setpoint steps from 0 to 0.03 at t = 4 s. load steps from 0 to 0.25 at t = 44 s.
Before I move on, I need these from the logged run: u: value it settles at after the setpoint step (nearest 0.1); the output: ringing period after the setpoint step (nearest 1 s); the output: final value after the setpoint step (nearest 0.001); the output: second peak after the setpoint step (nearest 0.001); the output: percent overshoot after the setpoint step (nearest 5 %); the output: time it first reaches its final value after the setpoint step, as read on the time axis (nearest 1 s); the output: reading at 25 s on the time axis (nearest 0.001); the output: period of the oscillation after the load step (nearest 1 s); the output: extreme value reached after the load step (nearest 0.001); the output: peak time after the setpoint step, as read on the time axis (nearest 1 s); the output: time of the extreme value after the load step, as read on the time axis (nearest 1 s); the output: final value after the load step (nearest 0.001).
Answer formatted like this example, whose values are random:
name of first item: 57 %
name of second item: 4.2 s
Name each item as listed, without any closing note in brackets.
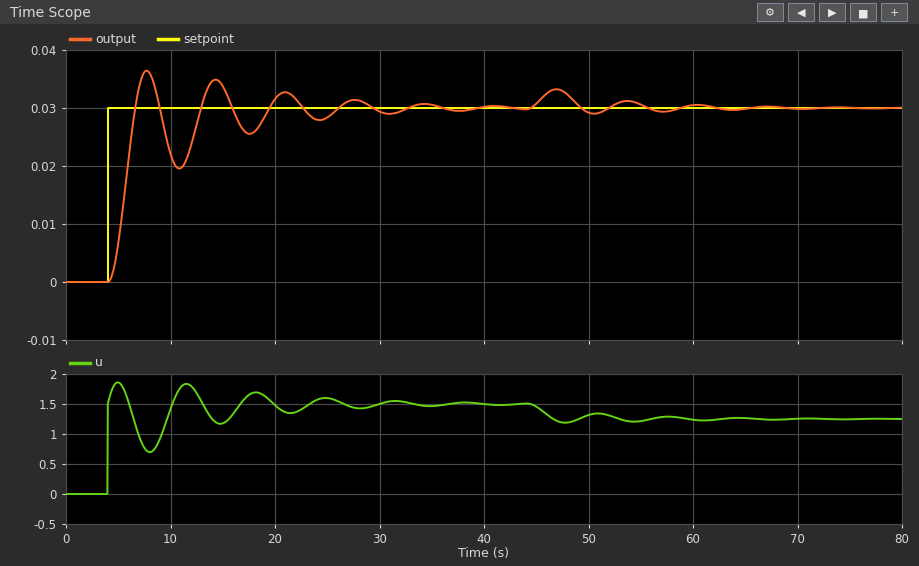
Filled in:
u: value it settles at after the setpoint step: 1.5
the output: ringing period after the setpoint step: 7 s
the output: final value after the setpoint step: 0.030
the output: second peak after the setpoint step: 0.035
the output: percent overshoot after the setpoint step: 20 %
the output: time it first reaches its final value after the setpoint step, as read on the time axis: 7 s
the output: reading at 25 s on the time axis: 0.028
the output: period of the oscillation after the load step: 7 s
the output: extreme value reached after the load step: 0.033
the output: peak time after the setpoint step, as read on the time axis: 8 s
the output: time of the extreme value after the load step, as read on the time axis: 47 s
the output: final value after the load step: 0.030
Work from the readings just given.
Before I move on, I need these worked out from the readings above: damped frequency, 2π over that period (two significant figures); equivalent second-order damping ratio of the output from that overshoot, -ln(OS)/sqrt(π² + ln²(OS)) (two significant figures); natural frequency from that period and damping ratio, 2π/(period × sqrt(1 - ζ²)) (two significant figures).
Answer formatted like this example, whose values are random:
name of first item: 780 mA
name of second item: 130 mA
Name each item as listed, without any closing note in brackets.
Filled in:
damped frequency, 2π over that period: 0.90 rad/s
equivalent second-order damping ratio of the output from that overshoot, -ln(OS)/sqrt(π² + ln²(OS)): 0.46
natural frequency from that period and damping ratio, 2π/(period × sqrt(1 - ζ²)): 1.0 rad/s
